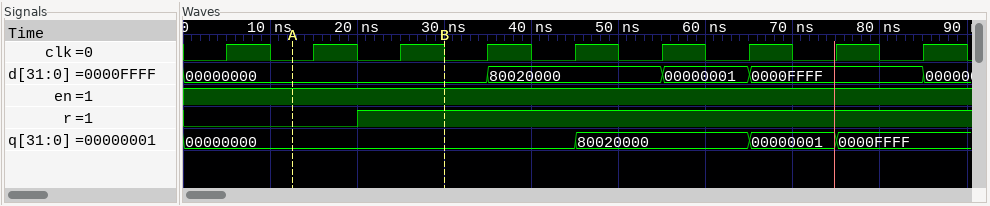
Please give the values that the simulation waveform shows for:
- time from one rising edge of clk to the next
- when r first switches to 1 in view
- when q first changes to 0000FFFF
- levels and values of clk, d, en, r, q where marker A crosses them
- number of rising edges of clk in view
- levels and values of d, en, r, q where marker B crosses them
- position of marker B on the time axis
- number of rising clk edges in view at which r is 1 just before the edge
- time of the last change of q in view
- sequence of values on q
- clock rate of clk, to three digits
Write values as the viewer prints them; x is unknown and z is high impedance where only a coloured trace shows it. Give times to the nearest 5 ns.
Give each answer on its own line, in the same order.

10 ns
20 ns
75 ns
clk=0, d=00000000, en=1, r=0, q=00000000
9
d=00000000, en=1, r=1, q=00000000
30 ns
7
75 ns
00000000, 80020000, 00000001, 0000FFFF
100 MHz
